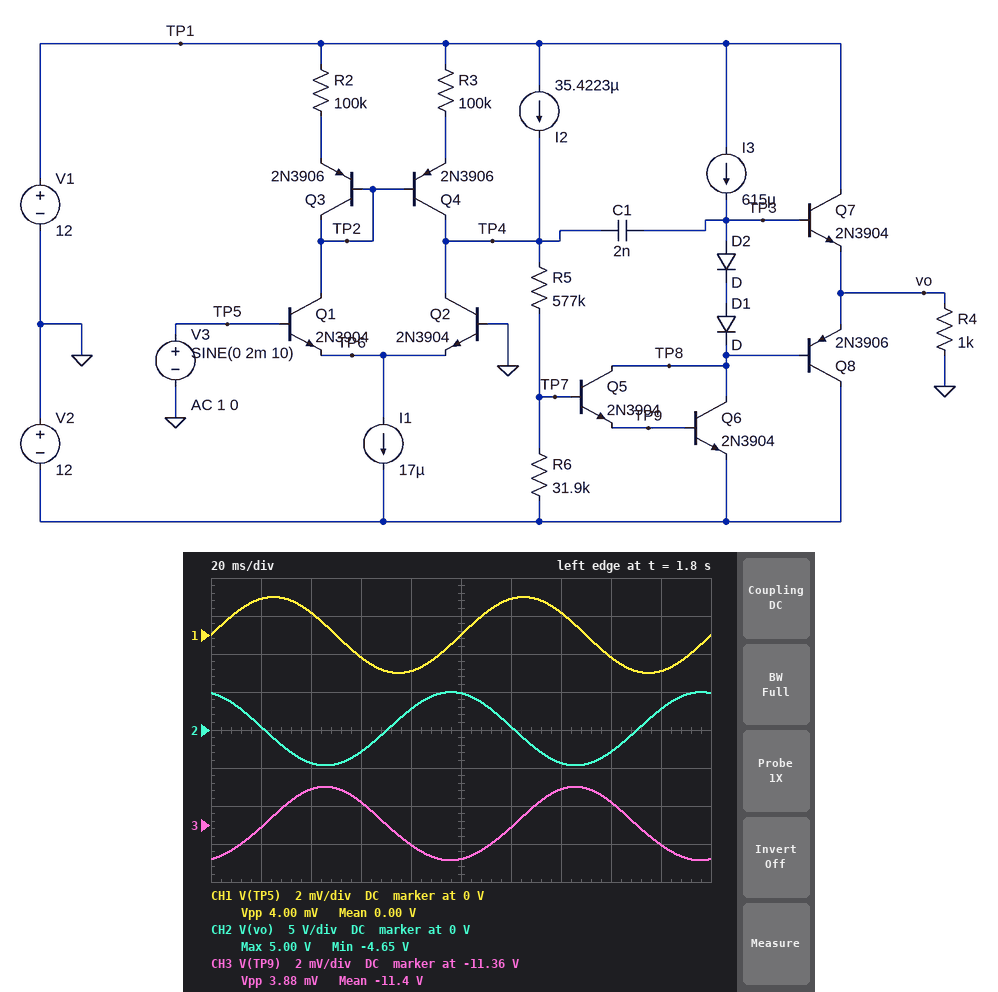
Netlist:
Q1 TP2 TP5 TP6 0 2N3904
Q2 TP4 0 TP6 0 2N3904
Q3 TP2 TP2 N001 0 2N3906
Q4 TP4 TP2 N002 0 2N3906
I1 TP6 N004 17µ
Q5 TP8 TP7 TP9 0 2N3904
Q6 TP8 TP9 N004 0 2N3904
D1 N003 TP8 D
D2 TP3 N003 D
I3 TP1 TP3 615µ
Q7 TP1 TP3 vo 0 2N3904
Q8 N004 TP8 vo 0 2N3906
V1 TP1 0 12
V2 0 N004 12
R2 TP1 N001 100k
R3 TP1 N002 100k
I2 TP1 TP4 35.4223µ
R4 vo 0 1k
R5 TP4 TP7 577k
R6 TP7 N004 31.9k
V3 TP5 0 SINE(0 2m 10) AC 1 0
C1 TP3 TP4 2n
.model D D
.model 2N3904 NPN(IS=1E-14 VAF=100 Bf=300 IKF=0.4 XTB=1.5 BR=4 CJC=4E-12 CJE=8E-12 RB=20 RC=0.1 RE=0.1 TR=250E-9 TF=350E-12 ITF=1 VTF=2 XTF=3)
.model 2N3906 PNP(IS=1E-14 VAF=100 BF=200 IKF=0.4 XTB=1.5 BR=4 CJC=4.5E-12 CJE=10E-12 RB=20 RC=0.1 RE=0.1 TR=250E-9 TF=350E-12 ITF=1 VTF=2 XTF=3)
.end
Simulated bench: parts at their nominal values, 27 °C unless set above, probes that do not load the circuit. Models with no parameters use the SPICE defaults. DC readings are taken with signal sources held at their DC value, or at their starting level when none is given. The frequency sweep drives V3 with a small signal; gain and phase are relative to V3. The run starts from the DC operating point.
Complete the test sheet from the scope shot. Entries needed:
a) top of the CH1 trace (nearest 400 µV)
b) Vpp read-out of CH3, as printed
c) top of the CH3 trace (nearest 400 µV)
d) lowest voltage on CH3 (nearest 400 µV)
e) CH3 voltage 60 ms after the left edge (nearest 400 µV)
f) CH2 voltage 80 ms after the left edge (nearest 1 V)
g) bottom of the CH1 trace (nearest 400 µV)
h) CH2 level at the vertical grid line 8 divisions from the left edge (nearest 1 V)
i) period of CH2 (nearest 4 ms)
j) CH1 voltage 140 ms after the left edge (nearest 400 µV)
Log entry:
2.0 mV
3.88 mV
-11.3580 V
-11.3620 V
-11.3588 V
3 V
-2.0 mV
-3 V
100 ms
1.2 mV
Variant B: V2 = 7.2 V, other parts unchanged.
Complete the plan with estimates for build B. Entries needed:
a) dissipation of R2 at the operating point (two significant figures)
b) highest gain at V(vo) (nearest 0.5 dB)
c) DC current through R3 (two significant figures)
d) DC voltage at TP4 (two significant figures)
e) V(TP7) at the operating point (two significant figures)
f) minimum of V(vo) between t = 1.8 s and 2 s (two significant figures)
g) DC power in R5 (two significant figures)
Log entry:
3.8 µW
-56.0 dB
5.9 µA
11 V
-6.2 V
12 V
540 µW
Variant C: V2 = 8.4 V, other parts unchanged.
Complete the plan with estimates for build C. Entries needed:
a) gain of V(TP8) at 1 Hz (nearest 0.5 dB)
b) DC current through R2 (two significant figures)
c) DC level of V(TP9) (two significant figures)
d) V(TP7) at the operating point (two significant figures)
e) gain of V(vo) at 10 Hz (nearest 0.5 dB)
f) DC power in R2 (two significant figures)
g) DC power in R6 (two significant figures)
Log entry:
-18.0 dB
7.0 µA
-7.8 V
-7.4 V
-40.0 dB
4.9 µW
33 µW
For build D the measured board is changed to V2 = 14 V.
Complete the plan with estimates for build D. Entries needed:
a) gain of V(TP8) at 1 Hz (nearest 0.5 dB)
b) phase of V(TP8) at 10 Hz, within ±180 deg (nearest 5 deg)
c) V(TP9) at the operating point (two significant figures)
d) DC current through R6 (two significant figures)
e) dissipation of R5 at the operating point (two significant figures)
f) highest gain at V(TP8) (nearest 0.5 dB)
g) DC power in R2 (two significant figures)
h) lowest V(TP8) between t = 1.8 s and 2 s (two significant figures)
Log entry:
78.5 dB
105 deg
-13 V
36 µA
730 µW
79.0 dB
7.3 µW
-11 V
